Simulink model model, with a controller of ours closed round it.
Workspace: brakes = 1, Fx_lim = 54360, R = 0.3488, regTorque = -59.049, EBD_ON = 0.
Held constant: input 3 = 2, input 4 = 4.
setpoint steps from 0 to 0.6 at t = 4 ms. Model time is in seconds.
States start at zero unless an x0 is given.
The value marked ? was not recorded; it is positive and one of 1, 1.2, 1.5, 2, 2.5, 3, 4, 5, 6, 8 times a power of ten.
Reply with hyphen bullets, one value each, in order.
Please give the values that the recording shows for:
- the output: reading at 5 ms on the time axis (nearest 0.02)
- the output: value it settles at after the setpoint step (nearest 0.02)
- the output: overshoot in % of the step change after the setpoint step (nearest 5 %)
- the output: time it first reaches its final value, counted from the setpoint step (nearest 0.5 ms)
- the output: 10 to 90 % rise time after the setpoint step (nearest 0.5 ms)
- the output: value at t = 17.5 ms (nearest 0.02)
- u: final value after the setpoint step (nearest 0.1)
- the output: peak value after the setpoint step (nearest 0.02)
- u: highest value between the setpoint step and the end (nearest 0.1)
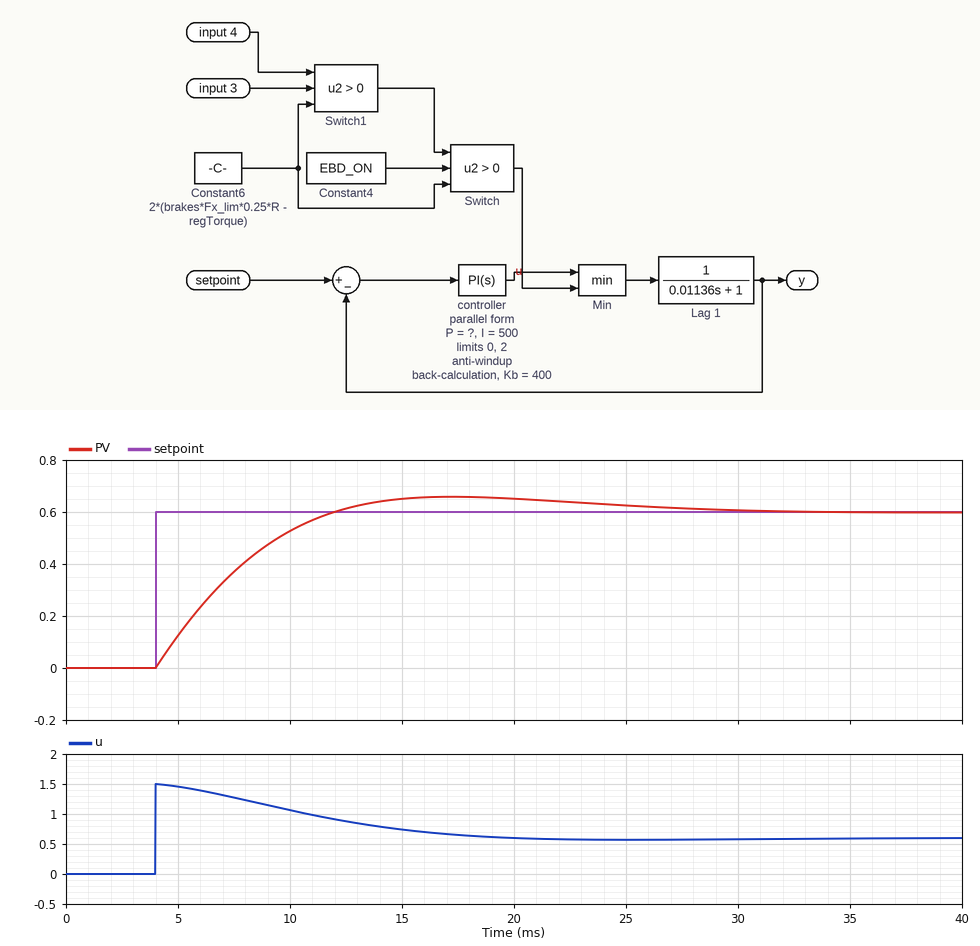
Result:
- 0.12
- 0.60
- 10 %
- 8.0 ms
- 6.0 ms
- 0.66
- 0.6
- 0.66
- 1.5
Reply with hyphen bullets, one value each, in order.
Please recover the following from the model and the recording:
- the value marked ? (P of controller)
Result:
- 2.5
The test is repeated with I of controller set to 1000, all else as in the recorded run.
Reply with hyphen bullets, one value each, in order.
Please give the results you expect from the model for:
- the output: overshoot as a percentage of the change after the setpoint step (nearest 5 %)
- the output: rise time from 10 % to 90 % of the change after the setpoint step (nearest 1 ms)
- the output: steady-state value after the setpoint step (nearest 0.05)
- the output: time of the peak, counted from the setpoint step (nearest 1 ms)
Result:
- 20 %
- 4 ms
- 0.60
- 9 ms
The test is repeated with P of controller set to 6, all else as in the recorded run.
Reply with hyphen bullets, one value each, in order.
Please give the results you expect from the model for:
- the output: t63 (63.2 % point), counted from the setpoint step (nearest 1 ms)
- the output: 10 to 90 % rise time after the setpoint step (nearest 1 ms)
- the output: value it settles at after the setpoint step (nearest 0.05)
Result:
- 3 ms
- 7 ms
- 0.60
